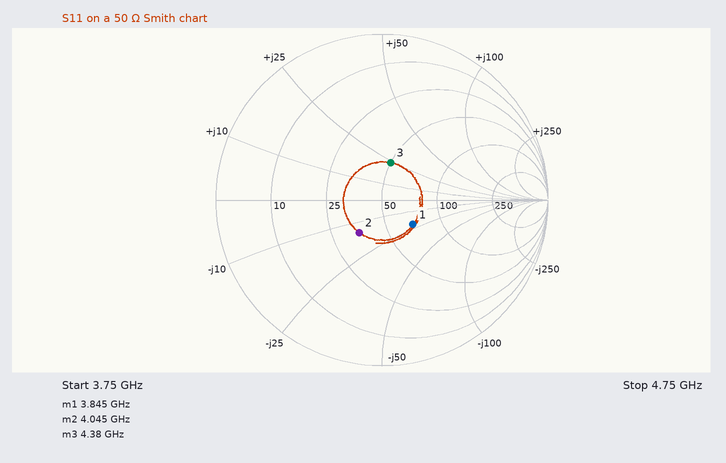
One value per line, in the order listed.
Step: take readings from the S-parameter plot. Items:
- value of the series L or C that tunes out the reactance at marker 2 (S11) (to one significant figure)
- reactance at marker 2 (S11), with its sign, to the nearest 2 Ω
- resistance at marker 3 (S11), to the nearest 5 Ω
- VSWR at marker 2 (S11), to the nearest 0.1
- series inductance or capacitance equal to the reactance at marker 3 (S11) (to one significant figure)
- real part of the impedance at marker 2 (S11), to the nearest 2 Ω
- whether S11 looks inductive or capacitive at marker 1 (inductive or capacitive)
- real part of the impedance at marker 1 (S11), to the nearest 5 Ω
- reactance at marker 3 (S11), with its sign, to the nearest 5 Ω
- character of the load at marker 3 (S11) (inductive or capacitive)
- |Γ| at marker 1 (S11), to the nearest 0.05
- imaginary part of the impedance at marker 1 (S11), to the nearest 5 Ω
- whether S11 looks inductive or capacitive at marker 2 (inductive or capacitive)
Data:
600 pH
-14 Ω
50 Ω
1.6
900 pH
36 Ω
capacitive
70 Ω
+25 Ω
inductive
0.25
-20 Ω
capacitive
